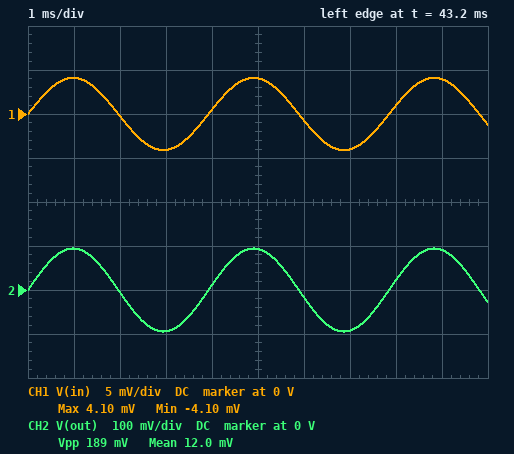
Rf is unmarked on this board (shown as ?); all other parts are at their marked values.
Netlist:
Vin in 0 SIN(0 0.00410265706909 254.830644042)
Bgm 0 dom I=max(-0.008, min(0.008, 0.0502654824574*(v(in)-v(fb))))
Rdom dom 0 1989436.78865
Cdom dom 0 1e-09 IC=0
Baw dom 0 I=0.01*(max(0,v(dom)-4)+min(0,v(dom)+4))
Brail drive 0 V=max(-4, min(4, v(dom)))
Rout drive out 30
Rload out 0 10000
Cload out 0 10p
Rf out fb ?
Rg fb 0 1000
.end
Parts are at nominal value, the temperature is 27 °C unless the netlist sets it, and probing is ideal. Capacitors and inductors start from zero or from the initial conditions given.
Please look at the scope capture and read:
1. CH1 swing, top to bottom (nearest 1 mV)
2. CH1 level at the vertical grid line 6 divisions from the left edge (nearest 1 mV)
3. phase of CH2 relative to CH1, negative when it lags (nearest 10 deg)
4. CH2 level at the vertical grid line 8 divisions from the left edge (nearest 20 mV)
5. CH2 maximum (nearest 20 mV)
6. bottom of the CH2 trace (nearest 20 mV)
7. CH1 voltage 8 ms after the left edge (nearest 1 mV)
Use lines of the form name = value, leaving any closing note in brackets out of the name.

CH1 swing, top to bottom = 8 mV
CH1 level at the vertical grid line 6 divisions from the left edge = -1 mV
phase of CH2 relative to CH1, negative when it lags = 0 deg
CH2 level at the vertical grid line 8 divisions from the left edge = 20 mV
CH2 maximum = 100 mV
bottom of the CH2 trace = -100 mV
CH1 voltage 8 ms after the left edge = 1 mV
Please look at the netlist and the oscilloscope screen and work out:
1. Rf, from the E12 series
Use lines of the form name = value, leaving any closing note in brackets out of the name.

Rf, from the E12 series = 22 kΩ
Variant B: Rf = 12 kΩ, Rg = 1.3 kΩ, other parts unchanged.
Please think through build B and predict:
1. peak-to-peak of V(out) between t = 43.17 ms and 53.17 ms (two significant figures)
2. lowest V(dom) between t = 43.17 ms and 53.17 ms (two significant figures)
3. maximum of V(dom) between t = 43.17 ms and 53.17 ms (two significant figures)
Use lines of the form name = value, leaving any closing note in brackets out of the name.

peak-to-peak of V(out) between t = 43.17 ms and 53.17 ms = 84 mV
lowest V(dom) between t = 43.17 ms and 53.17 ms = -42 mV
maximum of V(dom) between t = 43.17 ms and 53.17 ms = 42 mV
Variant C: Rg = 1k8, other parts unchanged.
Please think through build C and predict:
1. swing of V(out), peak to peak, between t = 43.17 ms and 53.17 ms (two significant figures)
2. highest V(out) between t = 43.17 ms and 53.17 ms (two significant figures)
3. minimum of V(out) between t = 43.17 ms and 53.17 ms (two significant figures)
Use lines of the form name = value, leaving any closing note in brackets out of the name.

swing of V(out), peak to peak, between t = 43.17 ms and 53.17 ms = 110 mV
highest V(out) between t = 43.17 ms and 53.17 ms = 54 mV
minimum of V(out) between t = 43.17 ms and 53.17 ms = -54 mV
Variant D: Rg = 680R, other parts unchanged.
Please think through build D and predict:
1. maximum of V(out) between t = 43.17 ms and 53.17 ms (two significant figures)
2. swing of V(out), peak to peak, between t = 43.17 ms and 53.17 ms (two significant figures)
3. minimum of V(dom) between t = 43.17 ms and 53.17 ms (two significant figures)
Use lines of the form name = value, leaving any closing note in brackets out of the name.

maximum of V(out) between t = 43.17 ms and 53.17 ms = 140 mV
swing of V(out), peak to peak, between t = 43.17 ms and 53.17 ms = 270 mV
minimum of V(dom) between t = 43.17 ms and 53.17 ms = -140 mV
